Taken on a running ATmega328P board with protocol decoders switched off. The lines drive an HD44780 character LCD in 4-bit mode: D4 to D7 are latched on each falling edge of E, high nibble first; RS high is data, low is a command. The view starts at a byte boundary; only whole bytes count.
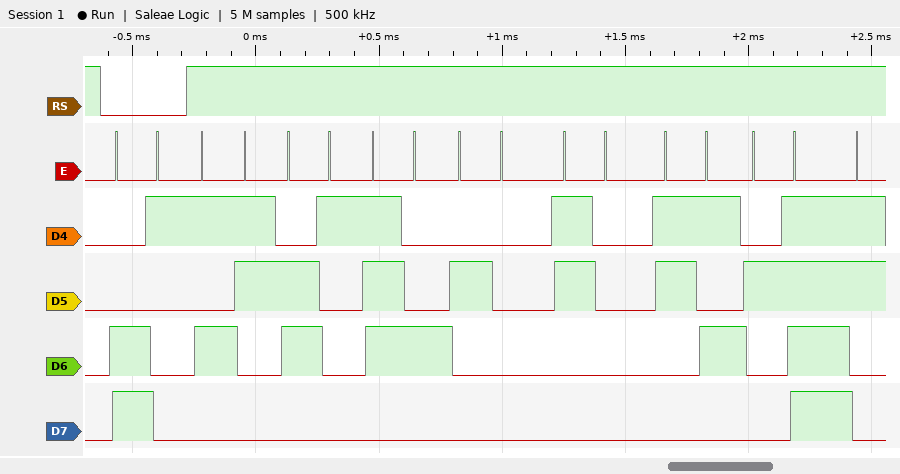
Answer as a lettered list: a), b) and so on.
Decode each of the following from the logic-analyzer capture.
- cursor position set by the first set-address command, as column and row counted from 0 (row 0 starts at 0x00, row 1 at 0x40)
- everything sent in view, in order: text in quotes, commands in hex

a) column 1, row 1
b) 0xC1 "Sat 05/"
